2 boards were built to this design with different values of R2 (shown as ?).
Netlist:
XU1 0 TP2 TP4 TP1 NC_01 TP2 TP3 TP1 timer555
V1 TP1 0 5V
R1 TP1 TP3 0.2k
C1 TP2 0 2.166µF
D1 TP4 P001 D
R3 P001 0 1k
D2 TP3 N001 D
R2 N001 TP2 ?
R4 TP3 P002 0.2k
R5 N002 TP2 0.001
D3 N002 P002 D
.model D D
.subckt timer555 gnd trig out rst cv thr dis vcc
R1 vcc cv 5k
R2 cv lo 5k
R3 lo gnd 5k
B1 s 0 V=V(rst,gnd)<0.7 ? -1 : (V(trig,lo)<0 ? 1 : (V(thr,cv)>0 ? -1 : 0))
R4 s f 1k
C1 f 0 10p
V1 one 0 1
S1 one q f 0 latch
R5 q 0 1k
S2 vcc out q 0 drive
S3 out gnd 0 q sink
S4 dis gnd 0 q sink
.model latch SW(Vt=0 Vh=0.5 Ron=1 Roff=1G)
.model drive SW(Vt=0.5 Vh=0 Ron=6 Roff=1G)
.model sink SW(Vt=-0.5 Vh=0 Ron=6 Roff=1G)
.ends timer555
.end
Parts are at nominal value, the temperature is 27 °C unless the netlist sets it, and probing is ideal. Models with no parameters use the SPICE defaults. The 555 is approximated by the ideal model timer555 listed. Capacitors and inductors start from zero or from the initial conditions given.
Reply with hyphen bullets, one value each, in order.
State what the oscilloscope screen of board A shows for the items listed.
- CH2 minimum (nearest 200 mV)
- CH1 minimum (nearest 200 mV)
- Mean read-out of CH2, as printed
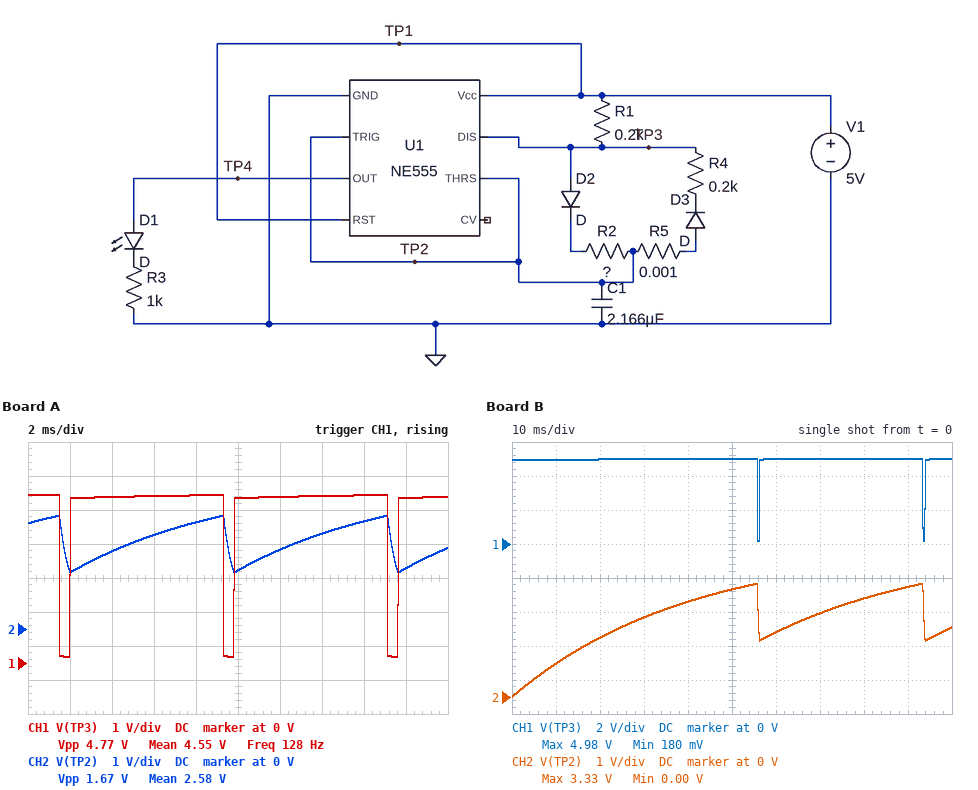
- 1.6 V
- 200 mV
- 2.58 V
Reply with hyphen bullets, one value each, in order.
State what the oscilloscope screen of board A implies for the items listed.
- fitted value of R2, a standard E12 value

- 3.3 kΩ
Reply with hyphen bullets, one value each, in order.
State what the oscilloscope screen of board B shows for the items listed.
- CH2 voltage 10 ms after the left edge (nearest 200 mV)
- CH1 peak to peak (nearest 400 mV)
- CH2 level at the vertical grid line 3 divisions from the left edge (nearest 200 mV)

- 1.0 V
- 4.8 V
- 2.4 V
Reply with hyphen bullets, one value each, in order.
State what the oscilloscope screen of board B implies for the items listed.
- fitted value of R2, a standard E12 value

- 18 kΩ
